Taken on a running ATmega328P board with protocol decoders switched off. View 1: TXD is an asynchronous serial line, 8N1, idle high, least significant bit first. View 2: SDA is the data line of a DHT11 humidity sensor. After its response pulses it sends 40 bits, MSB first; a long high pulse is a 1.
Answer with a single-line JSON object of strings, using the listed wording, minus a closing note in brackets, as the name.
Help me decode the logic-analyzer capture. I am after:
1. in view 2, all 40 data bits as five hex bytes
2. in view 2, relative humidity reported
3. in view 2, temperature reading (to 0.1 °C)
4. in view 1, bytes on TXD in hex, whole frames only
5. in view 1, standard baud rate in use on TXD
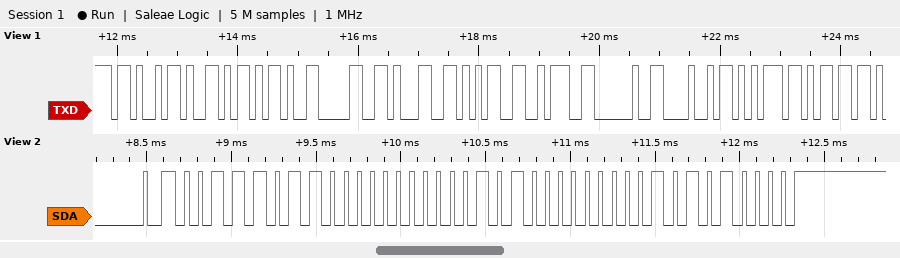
{"in view 2, all 40 data bits as five hex bytes": "3B 00 14 01 50", "in view 2, relative humidity reported": "59 %", "in view 2, temperature reading": "20.1 °C", "in view 1, bytes on TXD in hex, whole frames only": "4B 59 2D 30 31 35 3A 20 48 75 6D", "in view 1, standard baud rate in use on TXD": "9600 baud"}
